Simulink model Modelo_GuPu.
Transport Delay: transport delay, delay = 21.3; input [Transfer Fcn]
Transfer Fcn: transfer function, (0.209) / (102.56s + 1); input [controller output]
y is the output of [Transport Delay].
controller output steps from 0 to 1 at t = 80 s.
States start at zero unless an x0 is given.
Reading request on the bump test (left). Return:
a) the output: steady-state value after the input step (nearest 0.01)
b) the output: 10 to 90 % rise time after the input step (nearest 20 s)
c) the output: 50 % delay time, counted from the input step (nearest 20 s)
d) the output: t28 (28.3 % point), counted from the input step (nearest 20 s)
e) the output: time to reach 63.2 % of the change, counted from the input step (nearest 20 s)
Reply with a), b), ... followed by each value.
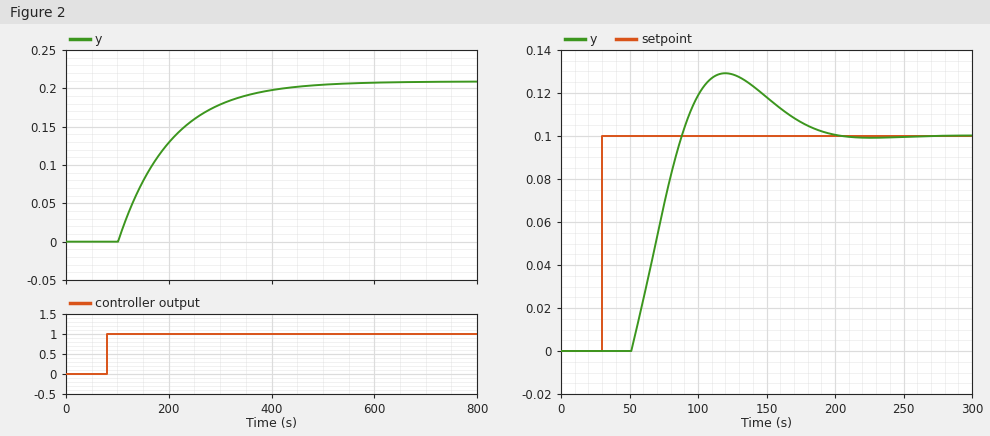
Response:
a) 0.21
b) 220 s
c) 100 s
d) 60 s
e) 120 s
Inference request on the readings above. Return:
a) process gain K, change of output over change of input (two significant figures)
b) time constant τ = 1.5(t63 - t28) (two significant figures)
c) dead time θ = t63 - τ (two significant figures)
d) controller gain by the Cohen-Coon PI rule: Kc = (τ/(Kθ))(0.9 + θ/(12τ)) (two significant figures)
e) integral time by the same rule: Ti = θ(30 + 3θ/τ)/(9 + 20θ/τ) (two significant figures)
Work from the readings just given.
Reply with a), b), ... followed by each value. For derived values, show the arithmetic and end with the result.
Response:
a) (0.21 - 0) / 1 = 0.21
b) 1.5 × (120 - 60) = 90 s
c) 120 - 90 = 30 s
d) 90 / (0.21 × 30) × (0.9 + 30 / (12 × 90)) = 13
e) 30 × (30 + 3 × 30 / 90) / (9 + 20 × 30 / 90) = 59 s
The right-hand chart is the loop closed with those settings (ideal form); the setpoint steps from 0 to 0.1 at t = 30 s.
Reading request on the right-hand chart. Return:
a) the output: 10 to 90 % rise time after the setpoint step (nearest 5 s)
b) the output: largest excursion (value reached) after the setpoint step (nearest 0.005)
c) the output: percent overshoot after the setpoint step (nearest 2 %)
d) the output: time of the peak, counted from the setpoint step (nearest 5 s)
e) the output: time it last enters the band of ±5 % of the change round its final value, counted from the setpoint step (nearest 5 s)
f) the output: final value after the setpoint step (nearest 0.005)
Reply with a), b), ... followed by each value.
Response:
a) 30 s
b) 0.130
c) 30 %
d) 90 s
e) 150 s
f) 0.100
